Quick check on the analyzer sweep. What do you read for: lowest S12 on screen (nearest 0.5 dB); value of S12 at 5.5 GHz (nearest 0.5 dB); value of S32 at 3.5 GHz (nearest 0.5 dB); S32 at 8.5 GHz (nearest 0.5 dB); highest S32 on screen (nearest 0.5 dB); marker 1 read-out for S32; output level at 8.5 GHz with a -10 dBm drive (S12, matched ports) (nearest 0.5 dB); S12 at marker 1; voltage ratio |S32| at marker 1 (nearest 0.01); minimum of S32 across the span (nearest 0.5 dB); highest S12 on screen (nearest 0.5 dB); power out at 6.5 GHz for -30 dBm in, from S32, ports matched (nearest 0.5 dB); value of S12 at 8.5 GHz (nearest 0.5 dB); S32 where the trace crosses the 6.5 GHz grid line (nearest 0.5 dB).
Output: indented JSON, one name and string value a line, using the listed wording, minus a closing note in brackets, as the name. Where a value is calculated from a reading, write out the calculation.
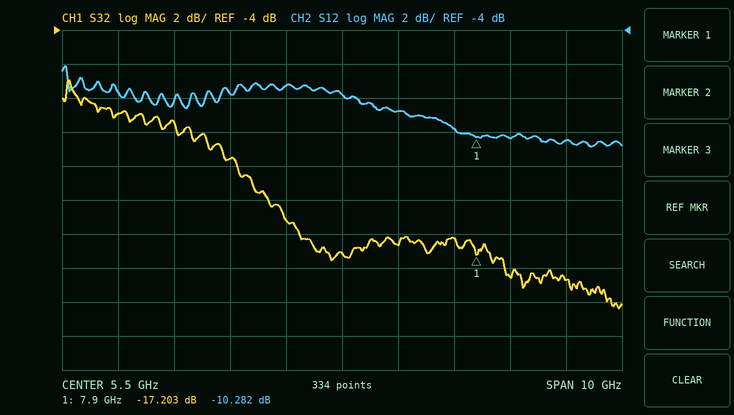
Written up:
{
  "lowest S12 on screen": "-11.0 dB",
  "value of S12 at 5.5 GHz": "-8.0 dB",
  "value of S32 at 3.5 GHz": "-11.5 dB",
  "S32 at 8.5 GHz": "-18.5 dB",
  "highest S32 on screen": "-7.0 dB",
  "marker 1 read-out for S32": "-17.203 dB",
  "output level at 8.5 GHz with a -10 dBm drive (S12, matched ports)": "-10 dBm + (-10.5 dB) = -20.5 dBm",
  "S12 at marker 1": "-10.282 dB",
  "voltage ratio |S32| at marker 1": "10^(-17.203/20) ≈ 0.14",
  "minimum of S32 across the span": "-20.5 dB",
  "highest S12 on screen": "-6.0 dB",
  "power out at 6.5 GHz for -30 dBm in, from S32, ports matched": "-30 dBm + (-16.5 dB) = -46.5 dBm",
  "value of S12 at 8.5 GHz": "-10.5 dB",
  "S32 where the trace crosses the 6.5 GHz grid line": "-16.5 dB"
}
